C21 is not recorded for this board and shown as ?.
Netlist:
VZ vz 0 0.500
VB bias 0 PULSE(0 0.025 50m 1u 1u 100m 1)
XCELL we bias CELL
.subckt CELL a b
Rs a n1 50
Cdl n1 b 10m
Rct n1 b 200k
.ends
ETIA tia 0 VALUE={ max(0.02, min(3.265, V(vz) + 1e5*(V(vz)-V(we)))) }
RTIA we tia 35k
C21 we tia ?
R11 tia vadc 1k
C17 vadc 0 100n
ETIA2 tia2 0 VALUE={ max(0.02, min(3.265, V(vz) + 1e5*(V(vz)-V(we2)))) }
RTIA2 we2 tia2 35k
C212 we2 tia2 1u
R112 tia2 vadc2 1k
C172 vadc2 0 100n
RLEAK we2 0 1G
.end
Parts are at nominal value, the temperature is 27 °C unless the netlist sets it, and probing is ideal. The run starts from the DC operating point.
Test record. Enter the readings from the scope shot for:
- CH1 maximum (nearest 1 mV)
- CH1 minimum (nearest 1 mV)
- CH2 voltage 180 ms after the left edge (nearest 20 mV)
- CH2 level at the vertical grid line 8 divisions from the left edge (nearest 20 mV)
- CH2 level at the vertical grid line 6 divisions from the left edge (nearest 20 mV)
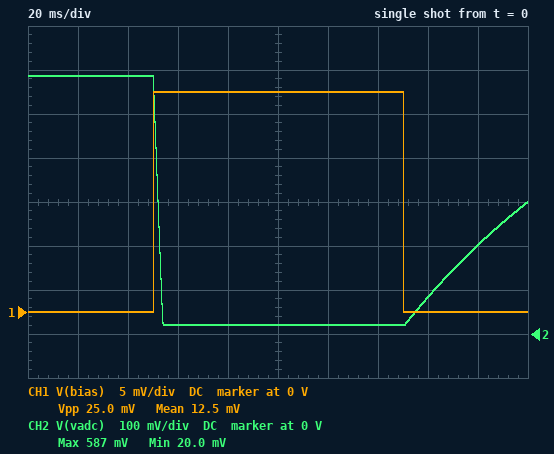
25 mV
0 V
200 mV
80 mV
20 mV
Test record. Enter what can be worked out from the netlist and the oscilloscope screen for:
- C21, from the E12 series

3.3 µF
